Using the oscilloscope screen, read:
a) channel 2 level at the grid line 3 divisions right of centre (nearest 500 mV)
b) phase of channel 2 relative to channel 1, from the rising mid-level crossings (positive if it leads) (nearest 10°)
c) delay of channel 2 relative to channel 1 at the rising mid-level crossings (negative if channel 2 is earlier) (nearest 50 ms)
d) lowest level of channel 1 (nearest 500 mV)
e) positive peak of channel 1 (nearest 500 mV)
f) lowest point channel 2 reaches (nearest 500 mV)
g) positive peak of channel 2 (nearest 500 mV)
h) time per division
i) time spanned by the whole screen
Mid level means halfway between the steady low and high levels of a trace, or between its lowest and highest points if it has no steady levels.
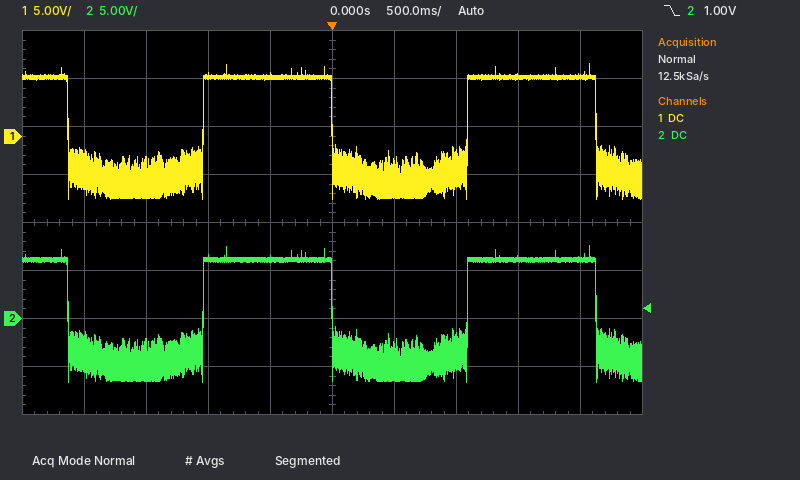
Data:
6.0 V
0°
0 ms
-6.5 V
7.5 V
-6.5 V
7.5 V
500 ms
5 s
